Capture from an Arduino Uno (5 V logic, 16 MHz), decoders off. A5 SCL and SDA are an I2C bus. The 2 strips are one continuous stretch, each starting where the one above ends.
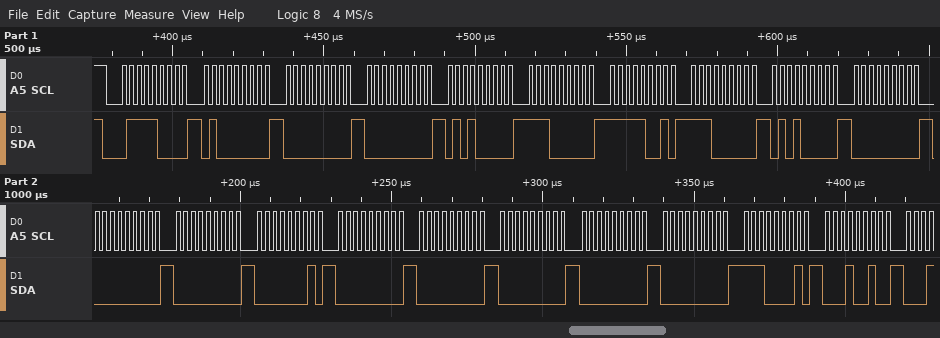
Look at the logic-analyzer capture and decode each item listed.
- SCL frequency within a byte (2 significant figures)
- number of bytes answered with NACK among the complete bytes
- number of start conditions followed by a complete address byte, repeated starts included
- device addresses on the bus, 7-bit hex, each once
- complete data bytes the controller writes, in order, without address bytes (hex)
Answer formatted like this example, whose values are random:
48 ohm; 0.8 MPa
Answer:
400 kHz; 0; 1; 0x3C; 40 00 00 50 E0 F9 E0 50 00 00 00 01 00 00 00 00 00 E1 12
